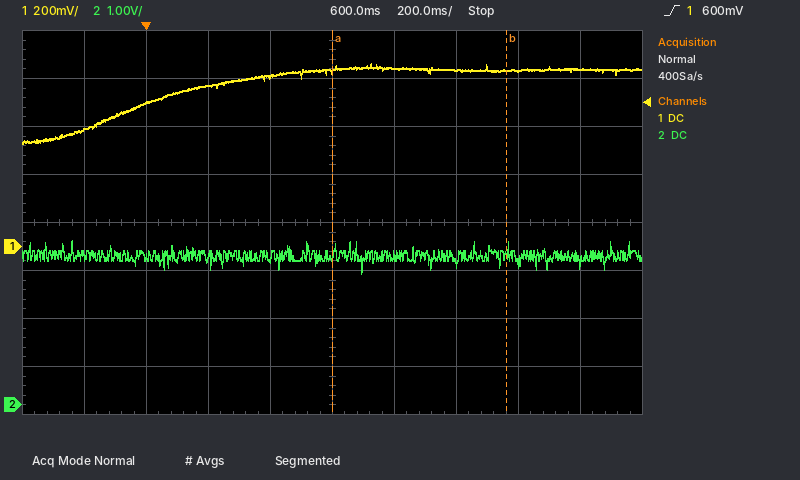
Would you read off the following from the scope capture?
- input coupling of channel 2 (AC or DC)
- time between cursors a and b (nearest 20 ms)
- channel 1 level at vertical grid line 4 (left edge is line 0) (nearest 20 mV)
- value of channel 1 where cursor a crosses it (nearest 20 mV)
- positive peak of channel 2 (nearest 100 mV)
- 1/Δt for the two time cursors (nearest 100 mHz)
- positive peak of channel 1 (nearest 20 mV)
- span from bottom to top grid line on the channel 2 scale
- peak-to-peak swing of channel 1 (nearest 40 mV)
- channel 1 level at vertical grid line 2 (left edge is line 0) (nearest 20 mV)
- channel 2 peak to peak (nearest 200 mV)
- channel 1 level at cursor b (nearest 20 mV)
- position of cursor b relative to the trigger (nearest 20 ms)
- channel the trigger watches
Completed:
DC
560 ms
700 mV
740 mV
3.4 V
1.8 Hz
760 mV
8 V
320 mV
600 mV
600 mV
740 mV
+1.16 s
channel 1
